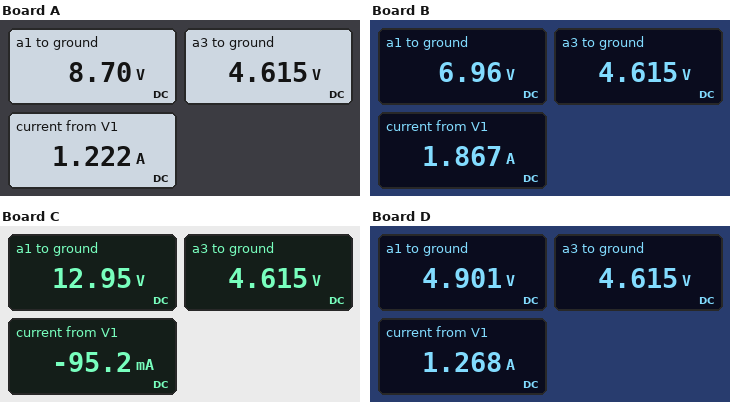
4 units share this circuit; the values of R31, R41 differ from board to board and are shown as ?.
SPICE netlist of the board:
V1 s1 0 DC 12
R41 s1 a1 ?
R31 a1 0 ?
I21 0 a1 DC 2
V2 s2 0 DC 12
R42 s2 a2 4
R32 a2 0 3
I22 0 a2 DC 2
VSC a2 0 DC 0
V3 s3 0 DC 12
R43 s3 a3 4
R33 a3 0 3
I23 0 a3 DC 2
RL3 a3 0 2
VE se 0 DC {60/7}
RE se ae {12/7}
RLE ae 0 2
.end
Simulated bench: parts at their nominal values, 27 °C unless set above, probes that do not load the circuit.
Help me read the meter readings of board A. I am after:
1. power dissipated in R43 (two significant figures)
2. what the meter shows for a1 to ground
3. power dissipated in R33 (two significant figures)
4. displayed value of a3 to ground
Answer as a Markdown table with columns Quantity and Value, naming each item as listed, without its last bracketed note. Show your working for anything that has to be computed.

| Quantity | Value |
|---|---|
| power dissipated in R43 | (12 V - 4.615 V)^2 / 4 Ω = 14 W |
| what the meter shows for a1 to ground | 8.70 V |
| power dissipated in R33 | (4.615 V)^2 / 3 Ω = 7.1 W |
| displayed value of a3 to ground | 4.615 V |
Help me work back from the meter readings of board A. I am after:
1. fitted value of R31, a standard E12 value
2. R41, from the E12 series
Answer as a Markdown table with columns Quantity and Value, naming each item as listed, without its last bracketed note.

| Quantity | Value |
|---|---|
| fitted value of R31, a standard E12 value | 2.7 Ω |
| R41, from the E12 series | 2.7 Ω |
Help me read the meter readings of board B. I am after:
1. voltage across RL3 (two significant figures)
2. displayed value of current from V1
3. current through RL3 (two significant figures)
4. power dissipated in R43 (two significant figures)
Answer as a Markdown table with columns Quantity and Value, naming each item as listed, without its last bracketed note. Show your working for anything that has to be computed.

| Quantity | Value |
|---|---|
| voltage across RL3 | 4.615 V = 4.6 V |
| displayed value of current from V1 | 1.867 A |
| current through RL3 | (4.615 V) / 2 Ω = 2.3 A |
| power dissipated in R43 | (12 V - 4.615 V)^2 / 4 Ω = 14 W |
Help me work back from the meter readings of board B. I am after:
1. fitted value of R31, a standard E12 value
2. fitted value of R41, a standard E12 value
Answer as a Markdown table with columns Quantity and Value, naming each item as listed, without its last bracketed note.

| Quantity | Value |
|---|---|
| fitted value of R31, a standard E12 value | 1.8 Ω |
| fitted value of R41, a standard E12 value | 2.7 Ω |
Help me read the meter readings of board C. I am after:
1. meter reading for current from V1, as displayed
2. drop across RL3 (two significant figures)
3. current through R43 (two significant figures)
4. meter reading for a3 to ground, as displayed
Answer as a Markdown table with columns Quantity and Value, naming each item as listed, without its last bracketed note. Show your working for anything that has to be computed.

| Quantity | Value |
|---|---|
| meter reading for current from V1, as displayed | -95.2 mA |
| drop across RL3 | 4.615 V = 4.6 V |
| current through R43 | (12 V - 4.615 V) / 4 Ω = 1.8 A |
| meter reading for a3 to ground, as displayed | 4.615 V |
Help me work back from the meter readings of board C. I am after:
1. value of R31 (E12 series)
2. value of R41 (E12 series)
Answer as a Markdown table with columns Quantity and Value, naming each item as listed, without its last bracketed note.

| Quantity | Value |
|---|---|
| value of R31 | 6.8 Ω |
| value of R41 | 10 Ω |
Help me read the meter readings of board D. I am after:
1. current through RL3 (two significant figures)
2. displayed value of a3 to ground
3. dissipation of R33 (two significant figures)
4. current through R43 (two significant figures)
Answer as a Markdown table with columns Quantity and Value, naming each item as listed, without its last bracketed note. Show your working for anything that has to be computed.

| Quantity | Value |
|---|---|
| current through RL3 | (4.615 V) / 2 Ω = 2.3 A |
| displayed value of a3 to ground | 4.615 V |
| dissipation of R33 | (4.615 V)^2 / 3 Ω = 7.1 W |
| current through R43 | (12 V - 4.615 V) / 4 Ω = 1.8 A |
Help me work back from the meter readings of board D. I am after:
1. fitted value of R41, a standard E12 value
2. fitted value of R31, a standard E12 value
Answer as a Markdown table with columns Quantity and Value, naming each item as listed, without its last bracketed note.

| Quantity | Value |
|---|---|
| fitted value of R41, a standard E12 value | 5.6 Ω |
| fitted value of R31, a standard E12 value | 1.5 Ω |
